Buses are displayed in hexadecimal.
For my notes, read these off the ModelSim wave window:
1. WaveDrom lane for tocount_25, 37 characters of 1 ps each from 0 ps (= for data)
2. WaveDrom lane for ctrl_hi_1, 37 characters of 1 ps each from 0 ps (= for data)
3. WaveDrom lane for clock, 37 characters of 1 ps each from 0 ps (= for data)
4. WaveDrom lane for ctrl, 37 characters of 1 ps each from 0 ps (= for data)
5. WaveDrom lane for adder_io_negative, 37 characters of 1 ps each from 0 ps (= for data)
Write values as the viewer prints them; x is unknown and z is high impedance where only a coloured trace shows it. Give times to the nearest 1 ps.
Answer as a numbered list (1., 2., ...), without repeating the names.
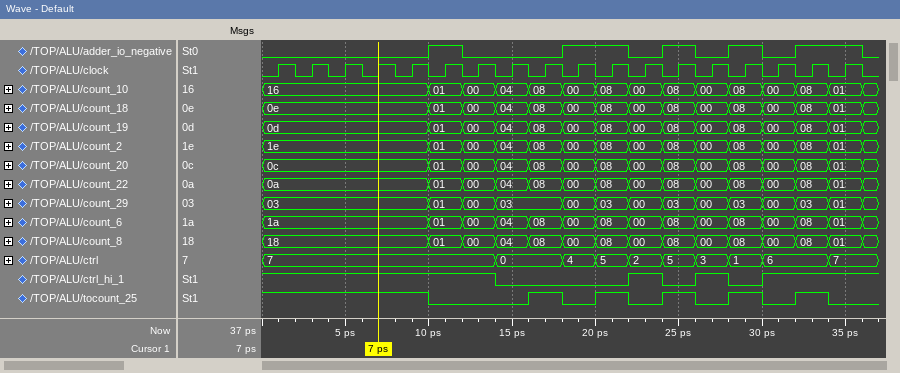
1. {name: 'tocount_25', wave: '1.........0.....1.0.1.0.1.0.1.0.1.0..'}
2. {name: 'ctrl_hi_1', wave: '1.............0.......1.0.1.0.1......'}
3. {name: 'clock', wave: '0101010101010101010101010101010101010'}
4. {name: 'ctrl', wave: '=.............=...=.=.=.=.=.=.=...=..', data: '7 0 4 5 2 5 3 1 6 7'}
5. {name: 'adder_io_negative', wave: '0.........1.0.....1...0.1.0.1.0.1...0'}
